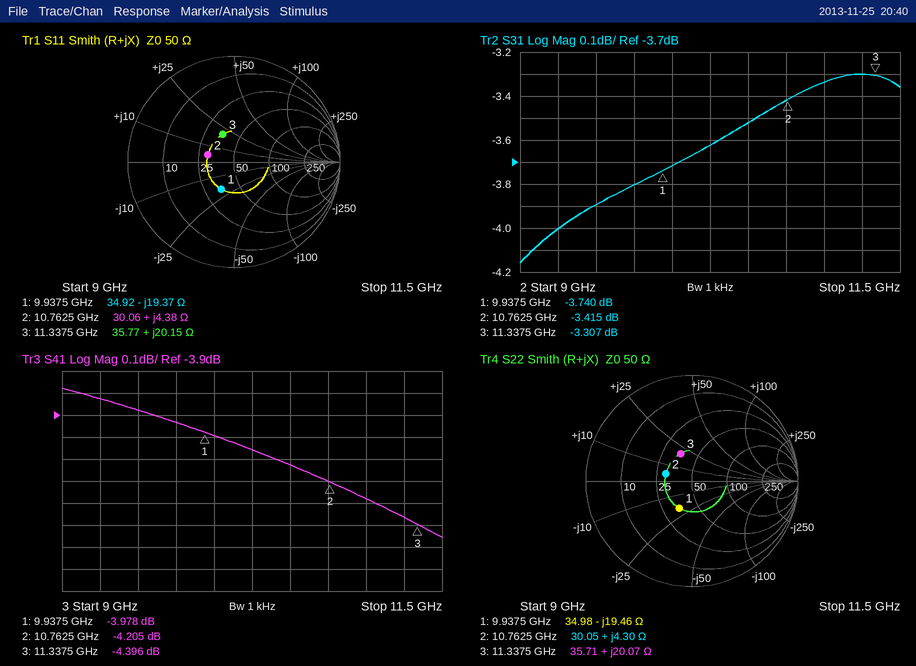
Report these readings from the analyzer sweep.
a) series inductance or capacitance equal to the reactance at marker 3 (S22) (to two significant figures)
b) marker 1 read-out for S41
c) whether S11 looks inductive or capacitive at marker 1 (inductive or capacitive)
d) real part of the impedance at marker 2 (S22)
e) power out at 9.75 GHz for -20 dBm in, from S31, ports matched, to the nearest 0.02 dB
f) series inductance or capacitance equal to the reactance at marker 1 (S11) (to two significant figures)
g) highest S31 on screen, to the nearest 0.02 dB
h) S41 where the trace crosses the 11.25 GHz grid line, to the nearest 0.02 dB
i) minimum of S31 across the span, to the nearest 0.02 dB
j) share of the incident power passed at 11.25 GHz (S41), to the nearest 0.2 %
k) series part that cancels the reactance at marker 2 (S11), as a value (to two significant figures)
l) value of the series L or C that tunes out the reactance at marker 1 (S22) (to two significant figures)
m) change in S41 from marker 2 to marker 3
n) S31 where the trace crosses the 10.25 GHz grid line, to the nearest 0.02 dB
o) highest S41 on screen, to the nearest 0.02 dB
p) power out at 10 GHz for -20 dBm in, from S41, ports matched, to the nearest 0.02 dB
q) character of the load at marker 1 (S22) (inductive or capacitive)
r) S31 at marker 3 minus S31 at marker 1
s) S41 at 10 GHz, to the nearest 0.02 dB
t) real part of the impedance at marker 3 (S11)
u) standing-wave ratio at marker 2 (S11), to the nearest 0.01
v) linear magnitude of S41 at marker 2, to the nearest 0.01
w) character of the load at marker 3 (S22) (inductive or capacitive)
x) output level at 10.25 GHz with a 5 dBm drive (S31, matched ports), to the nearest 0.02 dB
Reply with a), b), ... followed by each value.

a) 280 pH
b) -3.978 dB
c) capacitive
d) 30.05 Ω
e) -23.80 dBm
f) 830 fF
g) -3.30 dB
h) -4.36 dB
i) -4.16 dB
j) 36.6 %
k) 3.4 pF
l) 310 pH
m) -0.191 dB
n) -3.62 dB
o) -3.78 dB
p) -24.00 dBm
q) capacitive
r) 0.433 dB
s) -4.00 dB
t) 35.77 Ω
u) 1.68
v) 0.62
w) inductive
x) 1.38 dBm
